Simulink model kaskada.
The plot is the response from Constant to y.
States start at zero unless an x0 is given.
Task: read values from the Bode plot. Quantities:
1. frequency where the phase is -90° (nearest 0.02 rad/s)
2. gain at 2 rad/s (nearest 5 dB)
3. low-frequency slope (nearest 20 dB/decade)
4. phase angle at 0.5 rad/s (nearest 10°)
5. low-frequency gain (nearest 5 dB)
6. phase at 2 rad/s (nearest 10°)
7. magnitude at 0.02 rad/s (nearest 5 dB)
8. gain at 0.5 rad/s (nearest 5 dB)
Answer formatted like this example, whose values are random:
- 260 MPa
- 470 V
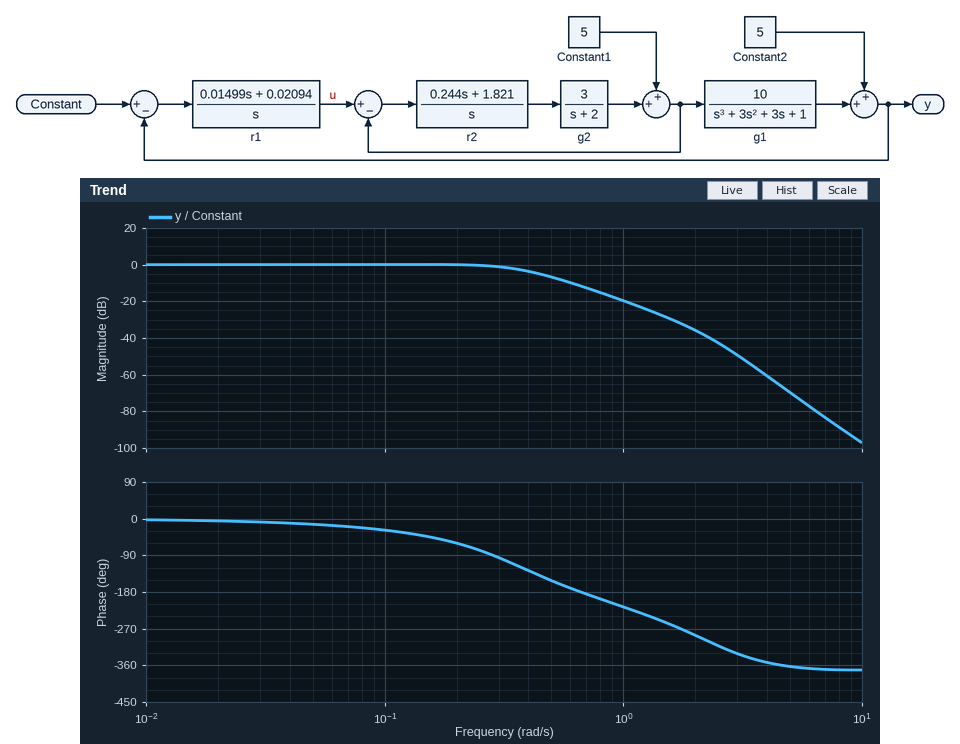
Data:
- 0.28 rad/s
- -35 dB
- 0 dB/decade
- -150°
- 0 dB
- -290°
- 0 dB
- -5 dB
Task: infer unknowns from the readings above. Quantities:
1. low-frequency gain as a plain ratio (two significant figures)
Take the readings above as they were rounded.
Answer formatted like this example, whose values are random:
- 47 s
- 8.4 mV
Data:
- 1.0
